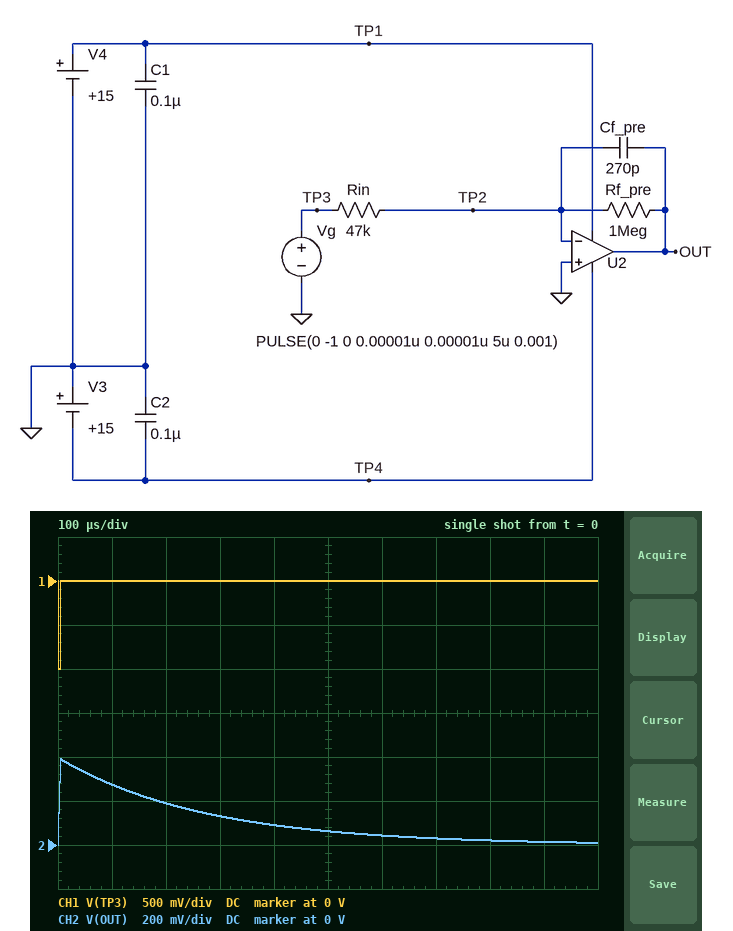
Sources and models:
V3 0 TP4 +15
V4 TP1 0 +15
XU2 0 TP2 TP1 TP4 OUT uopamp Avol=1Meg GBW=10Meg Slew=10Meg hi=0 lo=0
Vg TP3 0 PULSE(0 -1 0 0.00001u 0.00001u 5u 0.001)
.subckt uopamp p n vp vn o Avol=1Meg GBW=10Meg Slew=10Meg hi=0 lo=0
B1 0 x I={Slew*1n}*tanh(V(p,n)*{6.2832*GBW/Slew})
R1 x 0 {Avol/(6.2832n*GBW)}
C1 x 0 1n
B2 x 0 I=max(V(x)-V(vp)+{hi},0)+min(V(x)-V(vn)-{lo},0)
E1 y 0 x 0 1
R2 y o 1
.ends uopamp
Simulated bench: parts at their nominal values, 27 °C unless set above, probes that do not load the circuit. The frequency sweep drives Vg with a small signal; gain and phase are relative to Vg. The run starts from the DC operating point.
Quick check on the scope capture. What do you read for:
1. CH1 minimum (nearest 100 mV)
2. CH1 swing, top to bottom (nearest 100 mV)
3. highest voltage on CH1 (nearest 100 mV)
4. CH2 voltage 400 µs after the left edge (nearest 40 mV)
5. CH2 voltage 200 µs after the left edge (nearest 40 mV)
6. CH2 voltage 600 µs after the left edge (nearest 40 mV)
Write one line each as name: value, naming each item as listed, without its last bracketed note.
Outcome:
CH1 minimum: -1.0 V
CH1 swing, top to bottom: 1.0 V
highest voltage on CH1: 0 V
CH2 voltage 400 µs after the left edge: 80 mV
CH2 voltage 200 µs after the left edge: 200 mV
CH2 voltage 600 µs after the left edge: 40 mV
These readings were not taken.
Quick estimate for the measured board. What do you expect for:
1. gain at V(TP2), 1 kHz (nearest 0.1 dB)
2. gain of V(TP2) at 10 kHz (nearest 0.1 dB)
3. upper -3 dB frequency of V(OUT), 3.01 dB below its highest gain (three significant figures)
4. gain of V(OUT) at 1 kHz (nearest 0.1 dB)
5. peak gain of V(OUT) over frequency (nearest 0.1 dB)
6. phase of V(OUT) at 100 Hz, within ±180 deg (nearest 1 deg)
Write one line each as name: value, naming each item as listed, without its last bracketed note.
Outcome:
gain at V(TP2), 1 kHz: -59.3 dB
gain of V(TP2) at 10 kHz: -58.1 dB
upper -3 dB frequency of V(OUT), 3.01 dB below its highest gain: 589 Hz
gain of V(OUT) at 1 kHz: 20.7 dB
peak gain of V(OUT) over frequency: 26.6 dB
phase of V(OUT) at 100 Hz, within ±180 deg: 170 deg
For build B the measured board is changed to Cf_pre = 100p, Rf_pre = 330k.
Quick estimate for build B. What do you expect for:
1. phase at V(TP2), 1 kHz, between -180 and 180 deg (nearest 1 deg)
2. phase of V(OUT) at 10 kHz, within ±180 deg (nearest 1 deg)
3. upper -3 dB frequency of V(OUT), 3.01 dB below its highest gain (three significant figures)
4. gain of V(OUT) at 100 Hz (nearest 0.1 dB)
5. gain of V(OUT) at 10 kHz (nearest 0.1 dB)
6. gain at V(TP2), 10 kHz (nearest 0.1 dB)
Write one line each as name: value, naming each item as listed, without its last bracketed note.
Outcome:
phase at V(TP2), 1 kHz, between -180 and 180 deg: 78 deg
phase of V(OUT) at 10 kHz, within ±180 deg: 116 deg
upper -3 dB frequency of V(OUT), 3.01 dB below its highest gain: 4.81 kHz
gain of V(OUT) at 100 Hz: 16.9 dB
gain of V(OUT) at 10 kHz: 9.7 dB
gain at V(TP2), 10 kHz: -50.3 dB
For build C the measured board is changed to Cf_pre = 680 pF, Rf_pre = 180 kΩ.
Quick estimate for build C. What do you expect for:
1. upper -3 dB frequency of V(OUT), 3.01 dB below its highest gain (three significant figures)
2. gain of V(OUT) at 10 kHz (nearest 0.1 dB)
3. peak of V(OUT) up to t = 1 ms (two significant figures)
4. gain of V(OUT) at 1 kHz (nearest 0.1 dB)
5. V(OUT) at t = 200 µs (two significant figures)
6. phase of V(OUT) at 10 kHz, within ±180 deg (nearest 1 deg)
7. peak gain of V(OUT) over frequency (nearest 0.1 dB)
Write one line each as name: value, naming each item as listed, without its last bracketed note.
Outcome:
upper -3 dB frequency of V(OUT), 3.01 dB below its highest gain: 1.30 kHz
gain of V(OUT) at 10 kHz: -6.1 dB
peak of V(OUT) up to t = 1 ms: 150 mV
gain of V(OUT) at 1 kHz: 9.6 dB
V(OUT) at t = 200 µs: 31 mV
phase of V(OUT) at 10 kHz, within ±180 deg: 97 deg
peak gain of V(OUT) over frequency: 11.7 dB
